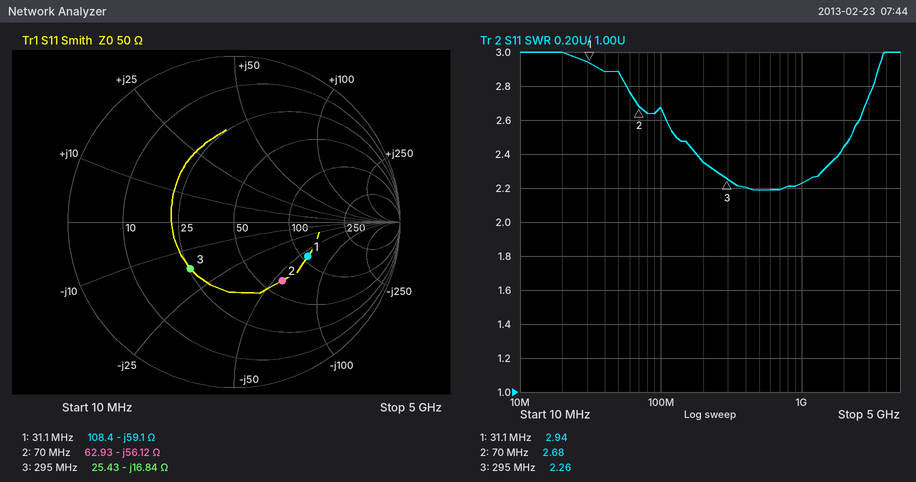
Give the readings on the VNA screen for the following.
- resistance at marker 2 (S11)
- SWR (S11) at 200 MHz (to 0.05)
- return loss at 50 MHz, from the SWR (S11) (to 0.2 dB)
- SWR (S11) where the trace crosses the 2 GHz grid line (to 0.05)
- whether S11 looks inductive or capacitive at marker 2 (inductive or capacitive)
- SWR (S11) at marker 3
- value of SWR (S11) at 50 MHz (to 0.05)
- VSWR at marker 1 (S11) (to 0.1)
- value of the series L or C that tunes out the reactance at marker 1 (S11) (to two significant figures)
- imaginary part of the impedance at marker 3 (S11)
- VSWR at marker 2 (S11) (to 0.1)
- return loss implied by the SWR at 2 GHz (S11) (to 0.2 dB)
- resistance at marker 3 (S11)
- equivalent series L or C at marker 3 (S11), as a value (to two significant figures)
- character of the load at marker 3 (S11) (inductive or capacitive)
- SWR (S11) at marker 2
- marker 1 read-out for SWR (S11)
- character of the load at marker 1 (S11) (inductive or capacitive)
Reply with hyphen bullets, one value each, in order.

- 62.93 Ω
- 2.35
- 6.2 dB
- 2.45
- capacitive
- 2.26
- 2.90
- 2.9
- 300 nH
- -16.84 Ω
- 2.7
- 7.6 dB
- 25.43 Ω
- 32 pF
- capacitive
- 2.68
- 2.94
- capacitive
